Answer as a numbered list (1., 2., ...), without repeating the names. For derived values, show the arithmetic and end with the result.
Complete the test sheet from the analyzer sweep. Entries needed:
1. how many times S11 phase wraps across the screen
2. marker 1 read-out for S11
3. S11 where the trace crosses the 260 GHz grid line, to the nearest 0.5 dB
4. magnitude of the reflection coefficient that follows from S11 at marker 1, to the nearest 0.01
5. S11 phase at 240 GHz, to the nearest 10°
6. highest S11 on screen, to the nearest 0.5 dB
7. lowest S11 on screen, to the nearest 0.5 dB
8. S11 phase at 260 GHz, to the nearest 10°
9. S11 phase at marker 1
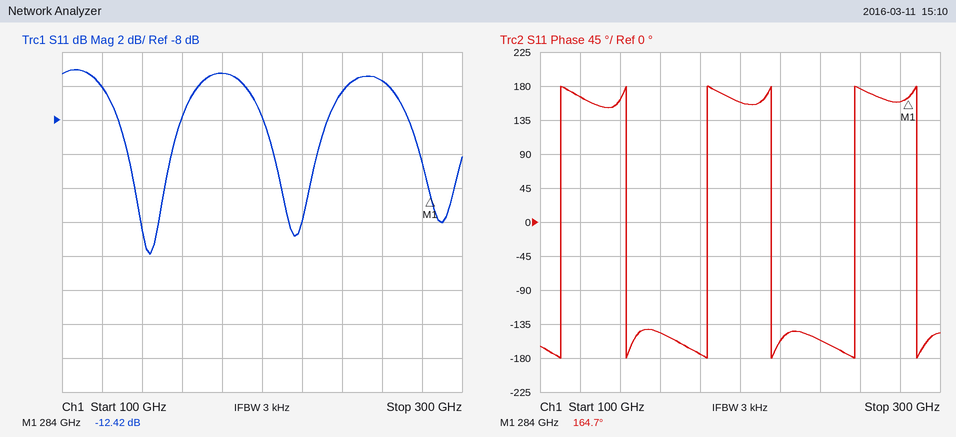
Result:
1. 6
2. -12.42 dB
3. -5.5 dB
4. 10^(-12.42/20) ≈ 0.24
5. -160°
6. -5.0 dB
7. -16.0 dB
8. 180°
9. 164.7°
